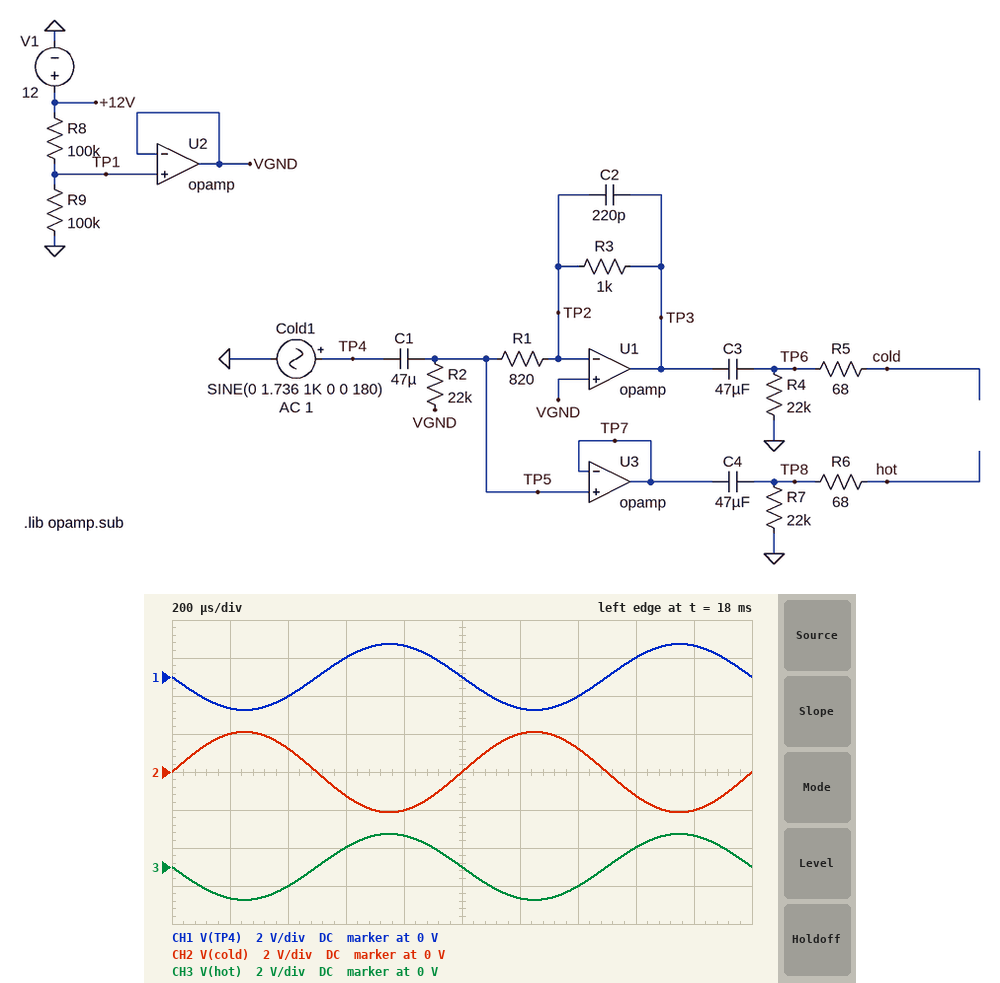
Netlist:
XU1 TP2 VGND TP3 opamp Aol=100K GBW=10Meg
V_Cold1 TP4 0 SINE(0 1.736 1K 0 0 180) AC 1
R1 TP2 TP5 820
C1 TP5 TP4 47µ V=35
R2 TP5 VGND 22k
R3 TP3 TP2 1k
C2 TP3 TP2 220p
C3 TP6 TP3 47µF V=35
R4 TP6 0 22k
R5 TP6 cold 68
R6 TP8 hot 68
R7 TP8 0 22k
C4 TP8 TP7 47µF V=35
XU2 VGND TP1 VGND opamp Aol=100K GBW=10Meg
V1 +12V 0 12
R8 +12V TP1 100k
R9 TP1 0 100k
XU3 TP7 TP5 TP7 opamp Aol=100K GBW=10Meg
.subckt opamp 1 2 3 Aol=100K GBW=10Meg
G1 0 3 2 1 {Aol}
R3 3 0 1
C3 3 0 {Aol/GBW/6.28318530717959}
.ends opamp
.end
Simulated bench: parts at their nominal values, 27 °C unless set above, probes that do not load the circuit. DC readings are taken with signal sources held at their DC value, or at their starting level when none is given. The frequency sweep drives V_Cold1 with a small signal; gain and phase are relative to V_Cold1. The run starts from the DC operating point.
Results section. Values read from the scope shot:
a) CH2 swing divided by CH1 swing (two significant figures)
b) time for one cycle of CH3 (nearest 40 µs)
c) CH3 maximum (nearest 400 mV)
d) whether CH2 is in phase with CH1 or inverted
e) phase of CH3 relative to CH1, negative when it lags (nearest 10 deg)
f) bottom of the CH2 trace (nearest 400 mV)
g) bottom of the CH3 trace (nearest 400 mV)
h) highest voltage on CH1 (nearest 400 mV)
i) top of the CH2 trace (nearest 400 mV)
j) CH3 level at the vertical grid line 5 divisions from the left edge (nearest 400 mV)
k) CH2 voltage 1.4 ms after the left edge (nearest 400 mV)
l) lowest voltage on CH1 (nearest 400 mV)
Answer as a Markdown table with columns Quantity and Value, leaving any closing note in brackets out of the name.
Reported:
| Quantity | Value |
|---|---|
| CH2 swing divided by CH1 swing | 1.2 |
| time for one cycle of CH3 | 1.00 ms |
| CH3 maximum | 1.6 V |
| whether CH2 is in phase with CH1 or inverted | inverted |
| phase of CH3 relative to CH1, negative when it lags | 0 deg |
| bottom of the CH2 trace | -2.0 V |
| bottom of the CH3 trace | -1.6 V |
| highest voltage on CH1 | 1.6 V |
| top of the CH2 trace | 2.0 V |
| CH3 level at the vertical grid line 5 divisions from the left edge | 0 V |
| CH2 voltage 1.4 ms after the left edge | 1.2 V |
| lowest voltage on CH1 | -1.6 V |
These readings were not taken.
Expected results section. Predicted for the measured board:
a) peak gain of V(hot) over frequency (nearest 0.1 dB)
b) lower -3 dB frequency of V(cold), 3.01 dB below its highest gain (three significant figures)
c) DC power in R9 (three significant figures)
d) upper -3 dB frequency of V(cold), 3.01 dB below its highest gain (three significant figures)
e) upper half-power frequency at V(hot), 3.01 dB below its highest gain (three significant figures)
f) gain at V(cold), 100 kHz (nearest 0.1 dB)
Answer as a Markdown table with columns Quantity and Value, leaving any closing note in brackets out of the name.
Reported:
| Quantity | Value |
|---|---|
| peak gain of V(hot) over frequency | 0 dB |
| lower -3 dB frequency of V(cold), 3.01 dB below its highest gain | 4.29 Hz |
| DC power in R9 | 360 µW |
| upper -3 dB frequency of V(cold), 3.01 dB below its highest gain | 659 kHz |
| upper half-power frequency at V(hot), 3.01 dB below its highest gain | 10.0 MHz |
| gain at V(cold), 100 kHz | 1.6 dB |
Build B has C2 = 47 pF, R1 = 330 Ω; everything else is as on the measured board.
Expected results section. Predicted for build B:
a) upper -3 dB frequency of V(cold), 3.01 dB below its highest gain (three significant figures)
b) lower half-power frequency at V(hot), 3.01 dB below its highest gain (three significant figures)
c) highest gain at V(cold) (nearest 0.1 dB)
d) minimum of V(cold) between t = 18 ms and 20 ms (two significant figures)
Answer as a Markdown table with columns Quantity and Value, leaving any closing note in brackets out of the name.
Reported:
| Quantity | Value |
|---|---|
| upper -3 dB frequency of V(cold), 3.01 dB below its highest gain | 1.52 MHz |
| lower half-power frequency at V(hot), 3.01 dB below its highest gain | 10.4 Hz |
| highest gain at V(cold) | 9.6 dB |
| minimum of V(cold) between t = 18 ms and 20 ms | -5.3 V |
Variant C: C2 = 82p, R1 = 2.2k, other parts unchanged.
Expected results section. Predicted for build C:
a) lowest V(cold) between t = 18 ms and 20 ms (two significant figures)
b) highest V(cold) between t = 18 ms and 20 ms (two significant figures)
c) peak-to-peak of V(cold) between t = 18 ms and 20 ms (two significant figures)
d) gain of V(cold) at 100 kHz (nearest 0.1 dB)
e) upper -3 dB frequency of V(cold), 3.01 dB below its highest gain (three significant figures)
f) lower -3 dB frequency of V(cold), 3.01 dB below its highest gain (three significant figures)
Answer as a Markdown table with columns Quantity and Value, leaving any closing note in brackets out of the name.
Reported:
| Quantity | Value |
|---|---|
| lowest V(cold) between t = 18 ms and 20 ms | -790 mV |
| highest V(cold) between t = 18 ms and 20 ms | 790 mV |
| peak-to-peak of V(cold) between t = 18 ms and 20 ms | 1.6 V |
| gain of V(cold) at 100 kHz | -6.9 dB |
| upper -3 dB frequency of V(cold), 3.01 dB below its highest gain | 1.71 MHz |
| lower -3 dB frequency of V(cold), 3.01 dB below its highest gain | 1.71 Hz |
